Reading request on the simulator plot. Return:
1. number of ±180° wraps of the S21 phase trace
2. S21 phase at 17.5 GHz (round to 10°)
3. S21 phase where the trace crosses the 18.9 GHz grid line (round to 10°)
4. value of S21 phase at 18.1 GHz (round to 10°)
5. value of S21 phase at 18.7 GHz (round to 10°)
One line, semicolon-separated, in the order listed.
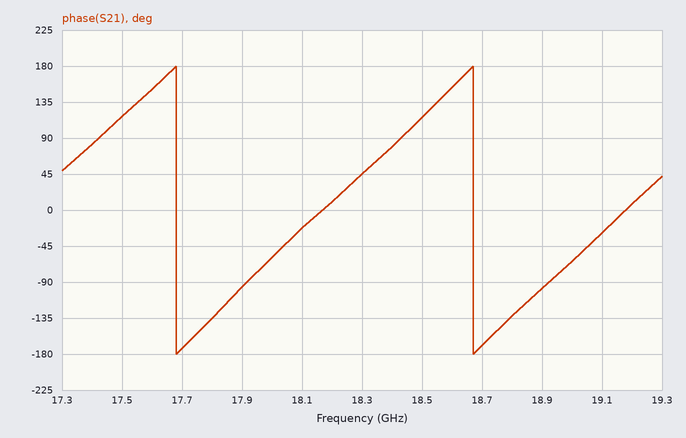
2; 120°; -100°; -20°; -170°
